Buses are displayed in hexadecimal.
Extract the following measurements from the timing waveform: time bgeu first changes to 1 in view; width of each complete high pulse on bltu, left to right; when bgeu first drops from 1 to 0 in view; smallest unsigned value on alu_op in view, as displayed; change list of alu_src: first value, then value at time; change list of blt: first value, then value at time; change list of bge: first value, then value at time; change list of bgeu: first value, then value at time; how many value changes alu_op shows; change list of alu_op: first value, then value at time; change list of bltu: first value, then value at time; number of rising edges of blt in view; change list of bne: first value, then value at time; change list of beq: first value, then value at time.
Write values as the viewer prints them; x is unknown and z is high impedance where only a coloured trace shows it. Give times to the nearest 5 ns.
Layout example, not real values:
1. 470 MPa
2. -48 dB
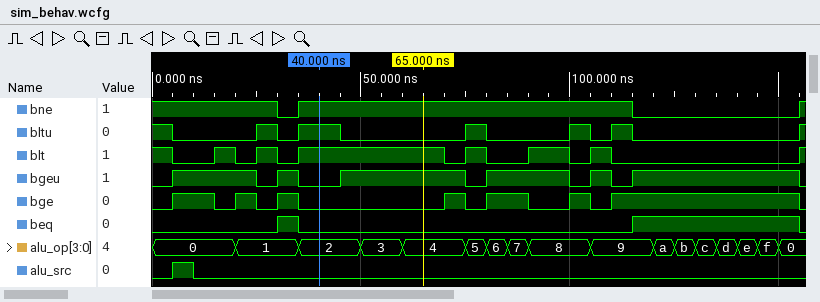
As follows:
1. 5 ns
2. 5 ns, 10 ns, 5 ns, 5 ns, 5 ns
3. 25 ns
4. 0
5. 0, 1 at 5 ns, 0 at 10 ns
6. 1, 0 at 5 ns, 1 at 15 ns, 0 at 20 ns, 1 at 25 ns, 0 at 30 ns, 1 at 35 ns, 0 at 70 ns, 1 at 75 ns, 0 at 80 ns, 1 at 90 ns, 0 at 100 ns, 1 at 105 ns, 0 at 110 ns, 1 at 155 ns
7. 0, 1 at 5 ns, 0 at 15 ns, 1 at 20 ns, 0 at 25 ns, 1 at 30 ns, 0 at 35 ns, 1 at 70 ns, 0 at 75 ns, 1 at 80 ns, 0 at 90 ns, 1 at 100 ns, 0 at 105 ns, 1 at 110 ns, 0 at 155 ns
8. 0, 1 at 5 ns, 0 at 25 ns, 1 at 30 ns, 0 at 35 ns, 1 at 45 ns, 0 at 75 ns, 1 at 80 ns, 0 at 100 ns, 1 at 105 ns, 0 at 110 ns, 1 at 115 ns, 0 at 155 ns
9. 16
10. 0, 1 at 20 ns, 2 at 35 ns, 3 at 50 ns, 4 at 60 ns, 5 at 75 ns, 6 at 80 ns, 7 at 85 ns, 8 at 90 ns, 9 at 105 ns, a at 120 ns, b at 125 ns, c at 130 ns, d at 135 ns, e at 140 ns, f at 145 ns, 0 at 150 ns
11. 1, 0 at 5 ns, 1 at 25 ns, 0 at 30 ns, 1 at 35 ns, 0 at 45 ns, 1 at 75 ns, 0 at 80 ns, 1 at 100 ns, 0 at 105 ns, 1 at 110 ns, 0 at 115 ns, 1 at 155 ns
12. 7
13. 1, 0 at 30 ns, 1 at 35 ns, 0 at 115 ns, 1 at 155 ns
14. 0, 1 at 30 ns, 0 at 35 ns, 1 at 115 ns, 0 at 155 ns
